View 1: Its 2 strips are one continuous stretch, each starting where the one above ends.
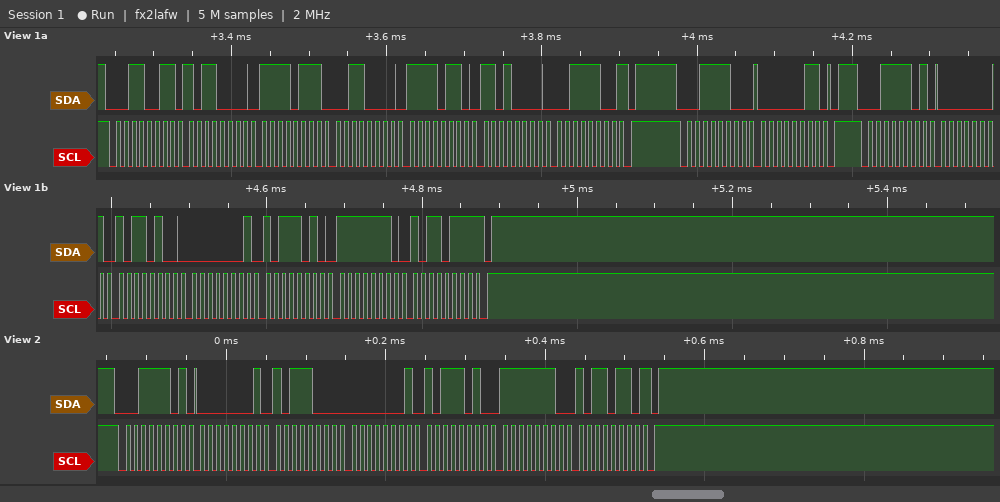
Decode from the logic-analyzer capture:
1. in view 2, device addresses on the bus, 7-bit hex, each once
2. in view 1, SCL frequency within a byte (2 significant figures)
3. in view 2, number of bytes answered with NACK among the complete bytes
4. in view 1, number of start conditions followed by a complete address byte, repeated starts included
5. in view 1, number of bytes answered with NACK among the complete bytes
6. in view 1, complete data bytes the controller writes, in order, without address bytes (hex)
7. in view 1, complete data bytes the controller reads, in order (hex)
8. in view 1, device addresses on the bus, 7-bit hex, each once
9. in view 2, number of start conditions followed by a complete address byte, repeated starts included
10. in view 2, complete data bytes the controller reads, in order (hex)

0x1E
100 kHz
1
3
2
03
B0 F7 30 F6 D0 3C 01 B4 01 BA FE B7
0x19 0x1E
1
01 B8 01 BA FE B6
